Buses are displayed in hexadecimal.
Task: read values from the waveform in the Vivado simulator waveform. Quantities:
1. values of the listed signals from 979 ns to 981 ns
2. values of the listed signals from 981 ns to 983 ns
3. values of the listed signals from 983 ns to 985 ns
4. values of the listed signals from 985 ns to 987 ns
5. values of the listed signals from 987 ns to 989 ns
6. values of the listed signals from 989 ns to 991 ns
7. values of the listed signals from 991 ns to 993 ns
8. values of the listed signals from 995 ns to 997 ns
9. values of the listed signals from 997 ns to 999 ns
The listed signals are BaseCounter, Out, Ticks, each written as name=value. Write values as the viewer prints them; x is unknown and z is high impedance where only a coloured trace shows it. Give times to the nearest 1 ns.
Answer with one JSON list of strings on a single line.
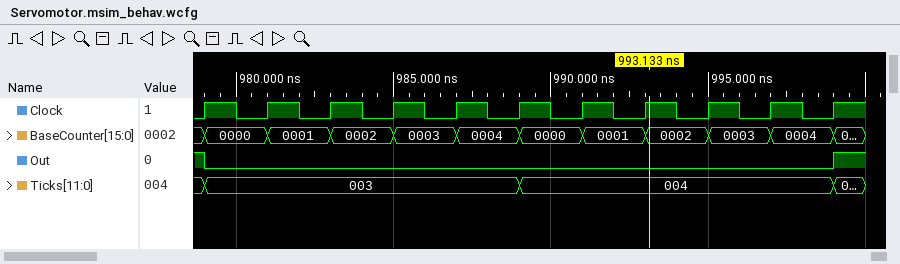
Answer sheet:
["BaseCounter=0000, Out=0, Ticks=003", "BaseCounter=0001, Out=0, Ticks=003", "BaseCounter=0002, Out=0, Ticks=003", "BaseCounter=0003, Out=0, Ticks=003", "BaseCounter=0004, Out=0, Ticks=003", "BaseCounter=0000, Out=0, Ticks=004", "BaseCounter=0001, Out=0, Ticks=004", "BaseCounter=0003, Out=0, Ticks=004", "BaseCounter=0004, Out=0, Ticks=004"]
